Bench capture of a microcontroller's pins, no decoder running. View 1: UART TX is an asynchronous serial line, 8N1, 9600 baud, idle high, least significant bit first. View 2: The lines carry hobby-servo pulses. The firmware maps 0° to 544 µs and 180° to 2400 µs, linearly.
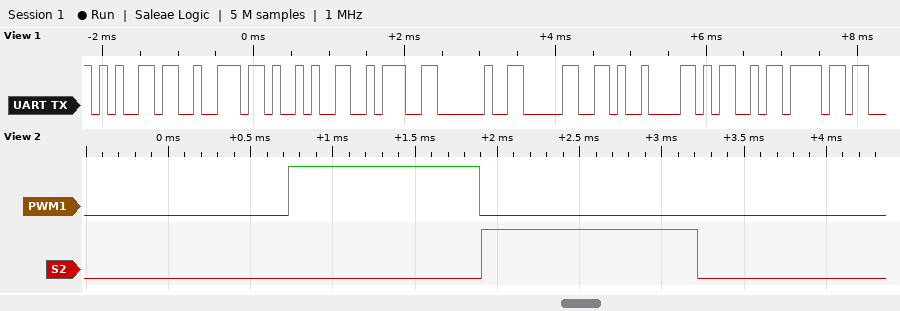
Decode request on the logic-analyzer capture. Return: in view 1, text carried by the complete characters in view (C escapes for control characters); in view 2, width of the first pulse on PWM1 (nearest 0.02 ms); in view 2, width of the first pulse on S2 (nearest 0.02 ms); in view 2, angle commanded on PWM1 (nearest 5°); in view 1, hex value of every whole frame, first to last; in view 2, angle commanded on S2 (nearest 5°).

"er): 0\tMo"
1.16 ms
1.32 ms
60°
65 72 29 3A 20 30 09 4D 6F
75°
